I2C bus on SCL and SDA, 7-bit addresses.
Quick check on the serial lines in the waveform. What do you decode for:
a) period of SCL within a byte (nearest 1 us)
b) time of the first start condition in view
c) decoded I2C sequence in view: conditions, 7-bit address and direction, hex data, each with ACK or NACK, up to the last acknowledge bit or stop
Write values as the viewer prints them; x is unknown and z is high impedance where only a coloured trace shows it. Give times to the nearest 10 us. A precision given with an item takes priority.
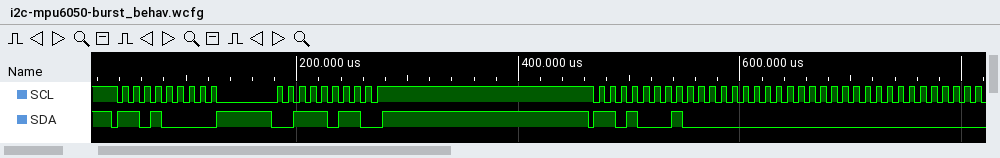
10 us
30 us
start, address 68 write ACK, 3B ACK, stop, start, address 68 read ACK, 00 ACK, 00 ACK
